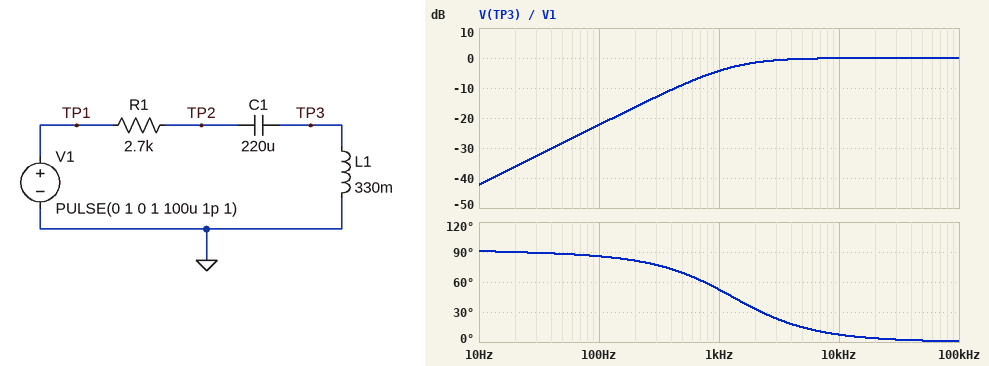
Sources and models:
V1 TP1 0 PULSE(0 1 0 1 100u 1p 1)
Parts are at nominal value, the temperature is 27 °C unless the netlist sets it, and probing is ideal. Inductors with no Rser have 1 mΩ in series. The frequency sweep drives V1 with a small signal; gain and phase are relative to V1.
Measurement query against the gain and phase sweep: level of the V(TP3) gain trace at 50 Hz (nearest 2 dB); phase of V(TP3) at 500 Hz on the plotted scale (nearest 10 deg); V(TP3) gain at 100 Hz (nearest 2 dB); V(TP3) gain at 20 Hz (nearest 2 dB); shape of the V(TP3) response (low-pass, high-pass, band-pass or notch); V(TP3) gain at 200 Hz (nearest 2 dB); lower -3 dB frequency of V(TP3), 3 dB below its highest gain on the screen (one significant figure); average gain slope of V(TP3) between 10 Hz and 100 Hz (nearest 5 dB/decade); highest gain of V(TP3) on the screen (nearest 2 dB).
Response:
-28 dB
70 deg
-22 dB
-36 dB
high-pass
-16 dB
1 kHz
20 dB/decade
0 dB
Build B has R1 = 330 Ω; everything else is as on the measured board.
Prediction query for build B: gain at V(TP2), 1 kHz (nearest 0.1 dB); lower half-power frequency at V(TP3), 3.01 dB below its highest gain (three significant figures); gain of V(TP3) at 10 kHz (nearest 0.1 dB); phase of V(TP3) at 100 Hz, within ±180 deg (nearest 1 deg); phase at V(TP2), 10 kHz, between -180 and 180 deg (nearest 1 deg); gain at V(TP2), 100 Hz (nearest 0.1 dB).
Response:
-0.1 dB
157 Hz
0 dB
59 deg
1 deg
-5.7 dB
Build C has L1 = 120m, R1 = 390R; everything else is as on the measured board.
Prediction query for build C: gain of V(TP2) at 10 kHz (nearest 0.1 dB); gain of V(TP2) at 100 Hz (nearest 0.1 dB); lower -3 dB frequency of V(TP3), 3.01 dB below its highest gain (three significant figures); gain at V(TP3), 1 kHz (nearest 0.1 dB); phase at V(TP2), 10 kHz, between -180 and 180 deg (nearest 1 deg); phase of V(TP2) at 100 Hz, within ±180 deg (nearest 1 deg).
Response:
0 dB
-15.3 dB
515 Hz
-1.0 dB
3 deg
80 deg
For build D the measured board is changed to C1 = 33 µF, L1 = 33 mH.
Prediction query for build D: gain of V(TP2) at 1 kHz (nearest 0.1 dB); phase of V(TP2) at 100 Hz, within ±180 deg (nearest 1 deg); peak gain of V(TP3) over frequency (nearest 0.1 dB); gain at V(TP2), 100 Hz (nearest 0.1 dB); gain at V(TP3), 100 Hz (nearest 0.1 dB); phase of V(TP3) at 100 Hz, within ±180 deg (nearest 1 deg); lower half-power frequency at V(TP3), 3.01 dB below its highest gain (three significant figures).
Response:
-22.5 dB
-89 deg
0 dB
-39.8 dB
-42.3 dB
91 deg
13.0 kHz
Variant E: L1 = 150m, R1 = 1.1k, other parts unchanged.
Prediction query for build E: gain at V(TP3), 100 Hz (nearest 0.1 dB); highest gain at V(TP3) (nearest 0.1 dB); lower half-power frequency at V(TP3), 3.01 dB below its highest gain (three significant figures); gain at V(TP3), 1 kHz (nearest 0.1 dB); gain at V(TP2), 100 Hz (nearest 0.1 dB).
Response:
-21.4 dB
0 dB
1.17 kHz
-3.7 dB
-22.1 dB
